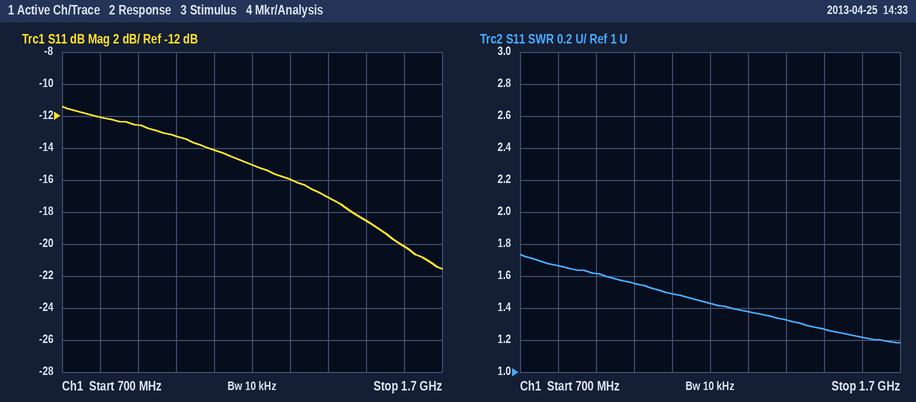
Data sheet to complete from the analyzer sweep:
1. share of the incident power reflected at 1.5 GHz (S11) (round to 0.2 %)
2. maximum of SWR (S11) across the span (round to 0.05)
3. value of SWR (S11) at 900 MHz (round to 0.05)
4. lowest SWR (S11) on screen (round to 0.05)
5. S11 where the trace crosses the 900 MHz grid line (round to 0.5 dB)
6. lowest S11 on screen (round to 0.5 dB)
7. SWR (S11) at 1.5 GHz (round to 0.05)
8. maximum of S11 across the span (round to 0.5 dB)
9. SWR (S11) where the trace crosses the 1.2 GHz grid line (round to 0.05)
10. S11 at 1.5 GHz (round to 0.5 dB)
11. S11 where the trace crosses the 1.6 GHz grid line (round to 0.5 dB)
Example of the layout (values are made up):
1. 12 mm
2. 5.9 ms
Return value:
1. 1.4 %
2. 1.75
3. 1.60
4. 1.20
5. -12.5 dB
6. -21.5 dB
7. 1.25
8. -11.5 dB
9. 1.45
10. -18.5 dB
11. -20.0 dB
